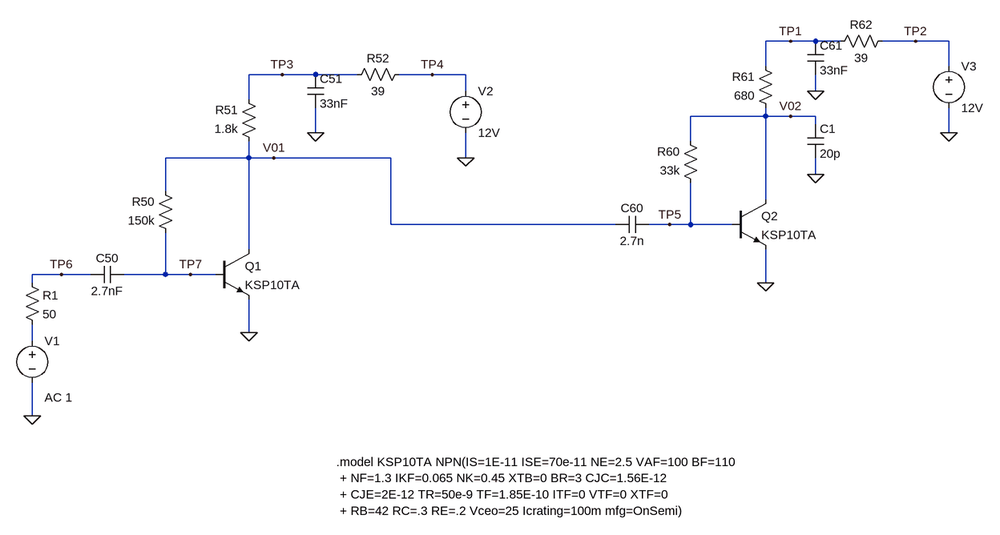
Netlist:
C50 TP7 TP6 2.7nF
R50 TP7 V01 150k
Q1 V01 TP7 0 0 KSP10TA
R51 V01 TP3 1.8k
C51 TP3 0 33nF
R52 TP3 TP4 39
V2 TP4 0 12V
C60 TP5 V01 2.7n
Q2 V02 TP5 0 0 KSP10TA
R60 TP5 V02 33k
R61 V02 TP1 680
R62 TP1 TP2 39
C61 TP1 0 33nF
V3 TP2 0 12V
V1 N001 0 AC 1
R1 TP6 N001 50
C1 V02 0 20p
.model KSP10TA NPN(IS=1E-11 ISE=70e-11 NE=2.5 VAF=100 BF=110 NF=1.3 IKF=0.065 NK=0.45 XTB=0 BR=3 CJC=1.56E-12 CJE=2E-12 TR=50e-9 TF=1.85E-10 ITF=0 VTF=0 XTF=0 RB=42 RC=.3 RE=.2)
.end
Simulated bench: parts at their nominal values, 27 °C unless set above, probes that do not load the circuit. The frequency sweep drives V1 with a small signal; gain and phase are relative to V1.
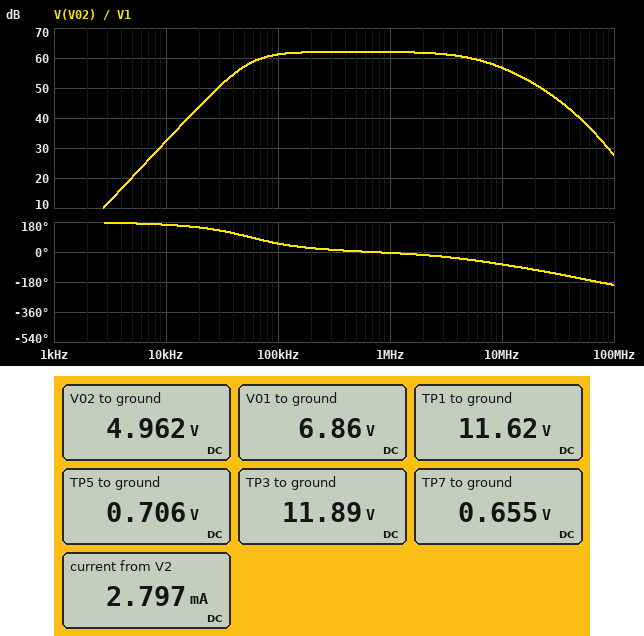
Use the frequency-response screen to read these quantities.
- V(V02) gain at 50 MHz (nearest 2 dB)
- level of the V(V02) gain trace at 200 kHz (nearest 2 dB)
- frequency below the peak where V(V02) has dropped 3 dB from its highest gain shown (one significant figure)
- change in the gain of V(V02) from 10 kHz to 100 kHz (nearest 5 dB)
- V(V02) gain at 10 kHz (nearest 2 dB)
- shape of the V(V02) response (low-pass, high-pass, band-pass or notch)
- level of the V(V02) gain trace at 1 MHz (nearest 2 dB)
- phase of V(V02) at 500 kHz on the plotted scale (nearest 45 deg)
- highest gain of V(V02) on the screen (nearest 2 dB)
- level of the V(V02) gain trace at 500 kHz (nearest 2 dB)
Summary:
40 dB
62 dB
60 kHz
30 dB
32 dB
band-pass
62 dB
0 deg
62 dB
62 dB
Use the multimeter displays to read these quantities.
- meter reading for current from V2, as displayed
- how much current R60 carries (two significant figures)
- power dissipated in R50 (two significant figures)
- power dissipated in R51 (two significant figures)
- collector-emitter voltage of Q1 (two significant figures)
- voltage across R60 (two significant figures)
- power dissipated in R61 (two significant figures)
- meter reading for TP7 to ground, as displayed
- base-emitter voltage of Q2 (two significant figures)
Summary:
2.797 mA
130 µA
260 µW
14 mW
6.9 V
4.3 V
65 mW
0.655 V
710 mV
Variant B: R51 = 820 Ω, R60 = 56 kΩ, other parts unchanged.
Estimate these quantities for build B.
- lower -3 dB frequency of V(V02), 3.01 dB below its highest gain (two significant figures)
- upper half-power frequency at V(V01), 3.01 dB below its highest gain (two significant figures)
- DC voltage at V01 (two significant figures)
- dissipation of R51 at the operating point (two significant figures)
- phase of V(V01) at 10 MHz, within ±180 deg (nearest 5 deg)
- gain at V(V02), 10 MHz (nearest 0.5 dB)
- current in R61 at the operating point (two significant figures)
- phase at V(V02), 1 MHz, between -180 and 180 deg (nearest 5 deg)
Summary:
92 kHz
220 kHz
8.7 V
12 mW
150 deg
59.0 dB
7.8 mA
-5 deg
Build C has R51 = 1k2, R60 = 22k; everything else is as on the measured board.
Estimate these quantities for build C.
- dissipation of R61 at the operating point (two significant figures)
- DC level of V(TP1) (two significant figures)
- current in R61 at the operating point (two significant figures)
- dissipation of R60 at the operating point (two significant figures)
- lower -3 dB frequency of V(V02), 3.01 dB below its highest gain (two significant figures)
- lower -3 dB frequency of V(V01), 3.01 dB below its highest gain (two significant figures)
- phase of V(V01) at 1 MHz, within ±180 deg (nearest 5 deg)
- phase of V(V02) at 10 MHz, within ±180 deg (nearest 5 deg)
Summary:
85 mW
12 V
11 mA
480 µW
79 kHz
32 kHz
155 deg
-70 deg
